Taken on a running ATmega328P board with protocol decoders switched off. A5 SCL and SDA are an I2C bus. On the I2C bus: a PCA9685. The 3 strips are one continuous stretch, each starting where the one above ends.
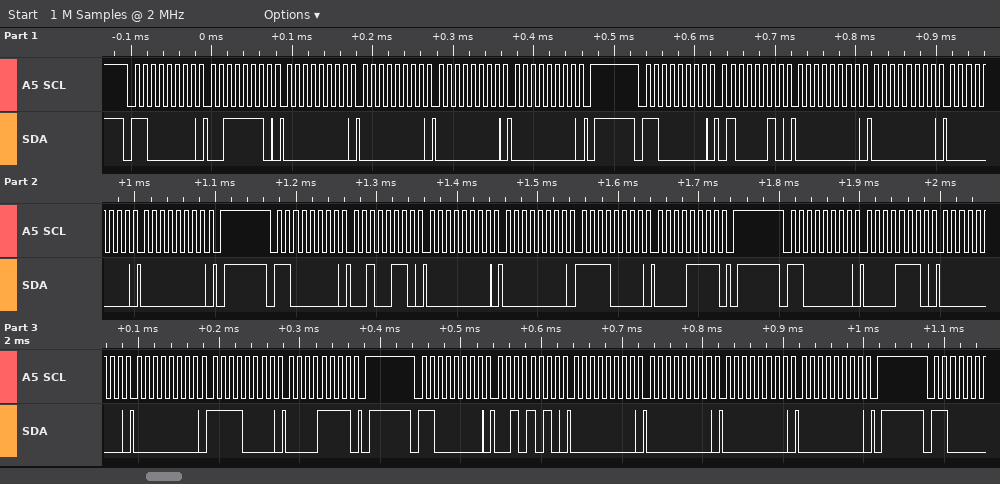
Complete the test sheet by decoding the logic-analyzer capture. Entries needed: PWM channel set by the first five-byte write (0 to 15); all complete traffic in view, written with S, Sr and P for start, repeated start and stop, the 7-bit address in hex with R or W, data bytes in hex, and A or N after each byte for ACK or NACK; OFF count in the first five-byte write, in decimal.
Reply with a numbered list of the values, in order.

1. 14
2. S 60W A 3E A 00 A 00 A 00 A 00 A P S 60W A 42 A 00 A 00 A 00 A 00 A P S 60W A 26 A 00 A 00 A F0 A 0F A P S 60W A 0E A 00 A 00 A F0 A 0F A P S 60W A 2A A 00 A 00 A 00 A 00 A P
3. 0
